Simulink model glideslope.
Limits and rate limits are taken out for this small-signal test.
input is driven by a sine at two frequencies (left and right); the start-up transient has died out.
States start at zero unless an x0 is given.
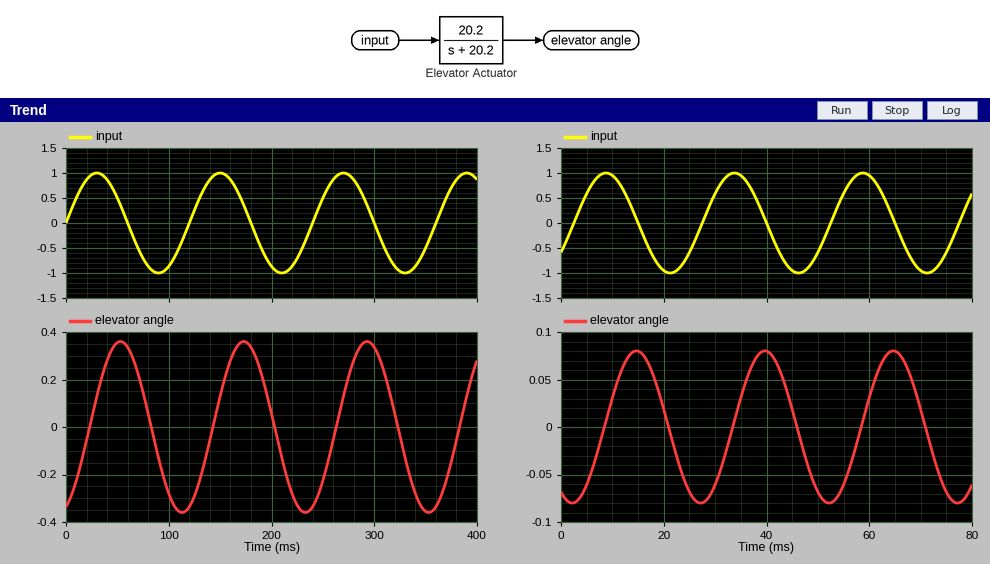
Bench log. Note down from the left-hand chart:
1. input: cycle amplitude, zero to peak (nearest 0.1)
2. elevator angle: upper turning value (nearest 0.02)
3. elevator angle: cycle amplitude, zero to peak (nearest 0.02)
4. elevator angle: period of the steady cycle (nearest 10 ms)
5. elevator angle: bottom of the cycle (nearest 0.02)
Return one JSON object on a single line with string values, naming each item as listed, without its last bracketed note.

{"input: cycle amplitude, zero to peak": "1.0", "elevator angle: upper turning value": "0.36", "elevator angle: cycle amplitude, zero to peak": "0.36", "elevator angle: period of the steady cycle": "120 ms", "elevator angle: bottom of the cycle": "-0.36"}
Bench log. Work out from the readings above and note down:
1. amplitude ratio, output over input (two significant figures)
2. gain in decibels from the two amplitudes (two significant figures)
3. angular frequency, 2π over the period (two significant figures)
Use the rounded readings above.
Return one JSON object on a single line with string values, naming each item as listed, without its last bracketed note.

{"amplitude ratio, output over input": "0.36", "gain in decibels from the two amplitudes": "-8.9 dB", "angular frequency, 2π over the period": "0.052 rad/ms"}
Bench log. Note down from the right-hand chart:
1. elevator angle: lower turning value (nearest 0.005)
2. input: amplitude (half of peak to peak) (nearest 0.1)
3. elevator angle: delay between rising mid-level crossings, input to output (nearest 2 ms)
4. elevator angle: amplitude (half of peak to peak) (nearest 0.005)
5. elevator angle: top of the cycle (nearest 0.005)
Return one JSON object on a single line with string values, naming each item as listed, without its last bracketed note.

{"elevator angle: lower turning value": "-0.080", "input: amplitude (half of peak to peak)": "1.0", "elevator angle: delay between rising mid-level crossings, input to output": "6 ms", "elevator angle: amplitude (half of peak to peak)": "0.080", "elevator angle: top of the cycle": "0.080"}
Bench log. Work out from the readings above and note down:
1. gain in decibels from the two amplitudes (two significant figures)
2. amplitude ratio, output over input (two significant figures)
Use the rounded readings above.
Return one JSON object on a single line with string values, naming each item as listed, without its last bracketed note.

{"gain in decibels from the two amplitudes": "-22 dB", "amplitude ratio, output over input": "0.080"}
